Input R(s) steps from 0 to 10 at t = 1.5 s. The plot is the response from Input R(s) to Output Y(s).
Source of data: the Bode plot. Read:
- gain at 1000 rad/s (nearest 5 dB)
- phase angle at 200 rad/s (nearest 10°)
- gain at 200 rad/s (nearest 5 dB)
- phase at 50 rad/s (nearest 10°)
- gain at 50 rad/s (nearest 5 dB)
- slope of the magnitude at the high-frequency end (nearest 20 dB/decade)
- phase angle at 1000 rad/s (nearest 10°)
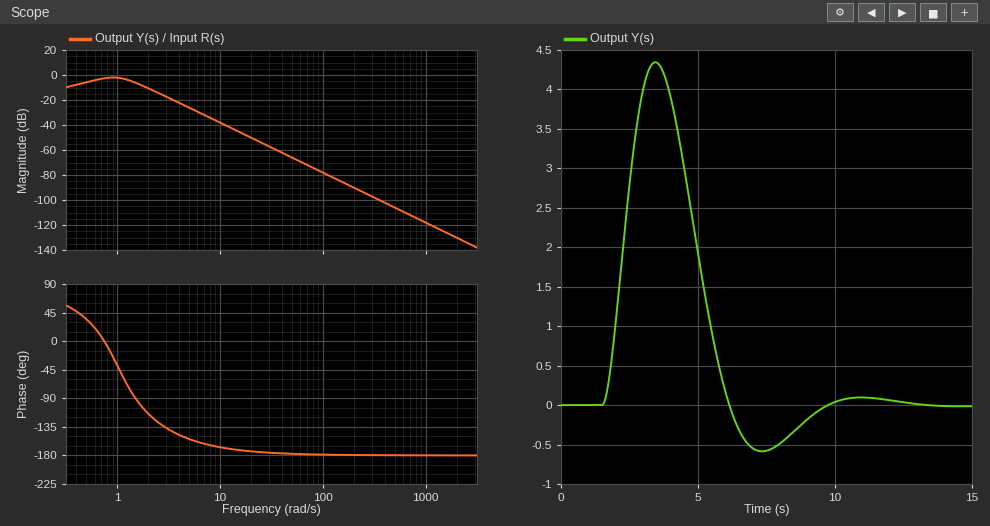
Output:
-120 dB
-180°
-90 dB
-180°
-65 dB
-40 dB/decade
-180°
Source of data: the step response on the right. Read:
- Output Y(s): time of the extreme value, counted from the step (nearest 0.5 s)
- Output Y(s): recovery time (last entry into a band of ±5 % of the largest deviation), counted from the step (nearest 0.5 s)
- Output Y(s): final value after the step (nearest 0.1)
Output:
2.0 s
7.5 s
0.0
